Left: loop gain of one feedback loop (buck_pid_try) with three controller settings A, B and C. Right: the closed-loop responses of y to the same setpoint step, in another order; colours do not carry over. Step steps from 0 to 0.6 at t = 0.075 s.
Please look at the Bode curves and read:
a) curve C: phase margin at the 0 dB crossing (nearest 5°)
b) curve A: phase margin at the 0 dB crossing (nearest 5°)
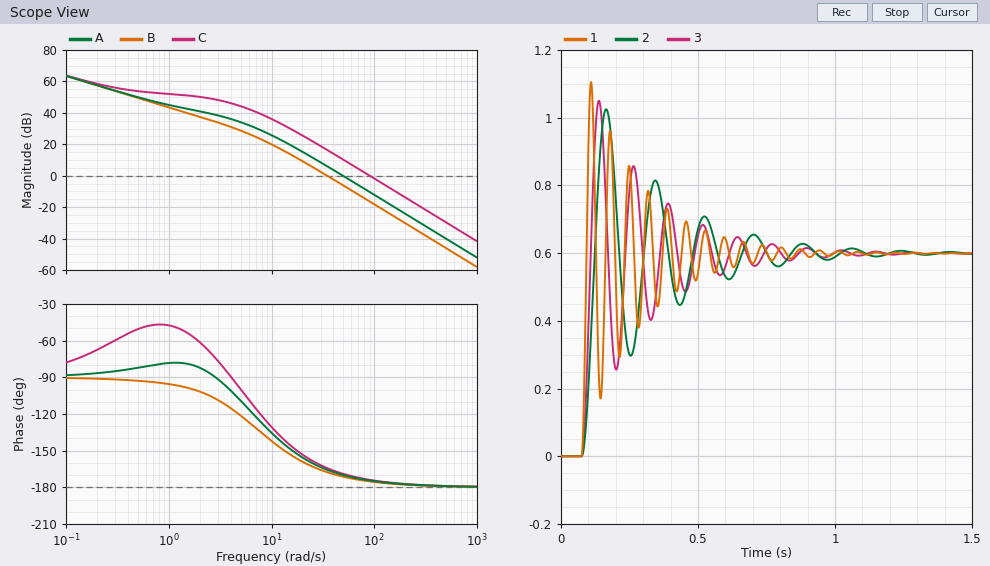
5°
10°
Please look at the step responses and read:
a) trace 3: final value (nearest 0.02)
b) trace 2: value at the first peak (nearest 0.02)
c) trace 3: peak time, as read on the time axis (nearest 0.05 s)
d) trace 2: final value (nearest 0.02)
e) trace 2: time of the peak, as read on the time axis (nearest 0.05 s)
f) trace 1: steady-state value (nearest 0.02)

0.60
1.02
0.15 s
0.60
0.15 s
0.60
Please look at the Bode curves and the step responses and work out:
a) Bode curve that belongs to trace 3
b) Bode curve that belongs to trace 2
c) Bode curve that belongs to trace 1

A
B
C
